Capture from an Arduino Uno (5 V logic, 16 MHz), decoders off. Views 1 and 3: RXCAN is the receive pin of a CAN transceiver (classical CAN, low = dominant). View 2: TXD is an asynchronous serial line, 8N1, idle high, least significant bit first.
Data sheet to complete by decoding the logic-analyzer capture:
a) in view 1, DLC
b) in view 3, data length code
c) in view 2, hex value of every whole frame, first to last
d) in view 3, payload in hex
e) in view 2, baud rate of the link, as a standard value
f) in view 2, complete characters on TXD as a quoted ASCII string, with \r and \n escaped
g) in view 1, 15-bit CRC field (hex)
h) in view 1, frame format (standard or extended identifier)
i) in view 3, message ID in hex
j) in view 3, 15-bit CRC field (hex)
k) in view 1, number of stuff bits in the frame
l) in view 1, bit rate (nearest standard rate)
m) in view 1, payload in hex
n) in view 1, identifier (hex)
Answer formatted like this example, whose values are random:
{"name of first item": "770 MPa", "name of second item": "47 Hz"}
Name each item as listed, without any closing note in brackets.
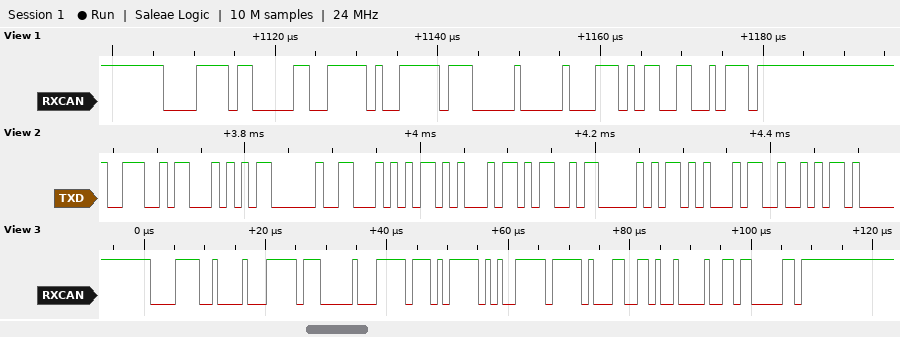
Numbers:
{"in view 1, DLC": "4", "in view 3, data length code": "8", "in view 2, hex value of every whole frame, first to last": "0x4E 0x54 0x20 0x54 0x45 0x4D 0x50 0x45 0x52", "in view 3, payload in hex": "FF 00 FF 5F A7 FF 19 A4", "in view 2, baud rate of the link, as a standard value": "115200 baud", "in view 2, complete characters on TXD as a quoted ASCII string, with \\r and \\n escaped": "\"NT TEMPER\"", "in view 1, 15-bit CRC field": "0x2CCB", "in view 1, frame format": "standard", "in view 3, message ID in hex": "0x0F2", "in view 3, 15-bit CRC field": "0x1360", "in view 1, number of stuff bits in the frame": "5", "in view 1, bit rate": "1000 kbit/s", "in view 1, payload in hex": "FC FF 00 07", "in view 1, identifier": "0x0F6"}
